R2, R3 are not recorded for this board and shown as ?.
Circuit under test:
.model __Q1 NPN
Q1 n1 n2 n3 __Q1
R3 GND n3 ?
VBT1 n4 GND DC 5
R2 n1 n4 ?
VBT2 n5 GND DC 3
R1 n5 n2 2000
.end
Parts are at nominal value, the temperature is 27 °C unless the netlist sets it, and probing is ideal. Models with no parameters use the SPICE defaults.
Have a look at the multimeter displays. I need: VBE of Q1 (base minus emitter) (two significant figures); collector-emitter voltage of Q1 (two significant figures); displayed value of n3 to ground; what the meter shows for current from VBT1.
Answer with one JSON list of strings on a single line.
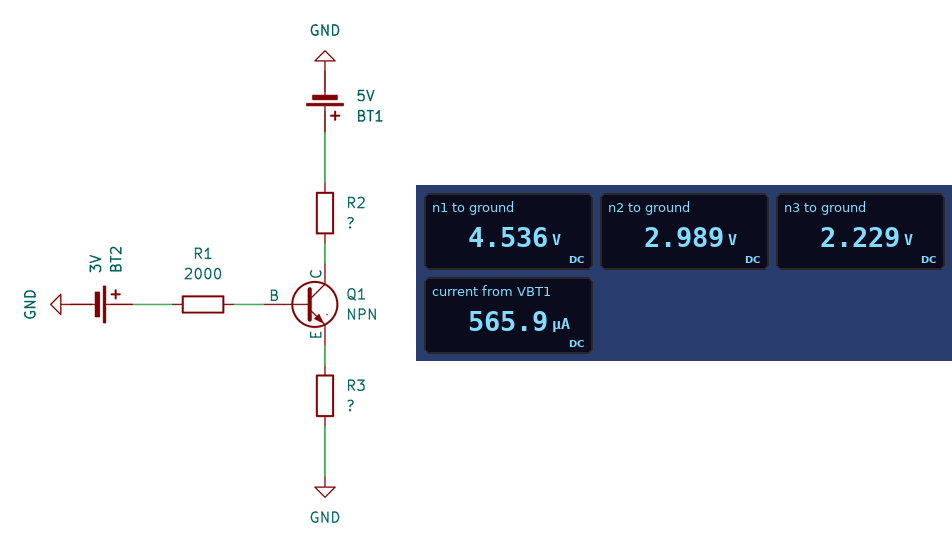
["760 mV", "2.3 V", "2.229 V", "565.9 µA"]
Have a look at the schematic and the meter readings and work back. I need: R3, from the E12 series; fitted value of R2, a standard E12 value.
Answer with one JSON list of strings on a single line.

["3.9 kΩ", "820 Ω"]
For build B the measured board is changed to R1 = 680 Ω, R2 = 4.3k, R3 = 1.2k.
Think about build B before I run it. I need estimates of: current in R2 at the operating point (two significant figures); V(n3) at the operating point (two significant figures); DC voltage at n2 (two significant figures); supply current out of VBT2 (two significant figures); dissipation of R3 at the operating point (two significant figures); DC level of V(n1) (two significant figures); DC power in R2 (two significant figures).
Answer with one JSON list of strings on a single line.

["750 µA", "1.7 V", "2.5 V", "690 µA", "2.5 mW", "1.8 V", "2.4 mW"]
